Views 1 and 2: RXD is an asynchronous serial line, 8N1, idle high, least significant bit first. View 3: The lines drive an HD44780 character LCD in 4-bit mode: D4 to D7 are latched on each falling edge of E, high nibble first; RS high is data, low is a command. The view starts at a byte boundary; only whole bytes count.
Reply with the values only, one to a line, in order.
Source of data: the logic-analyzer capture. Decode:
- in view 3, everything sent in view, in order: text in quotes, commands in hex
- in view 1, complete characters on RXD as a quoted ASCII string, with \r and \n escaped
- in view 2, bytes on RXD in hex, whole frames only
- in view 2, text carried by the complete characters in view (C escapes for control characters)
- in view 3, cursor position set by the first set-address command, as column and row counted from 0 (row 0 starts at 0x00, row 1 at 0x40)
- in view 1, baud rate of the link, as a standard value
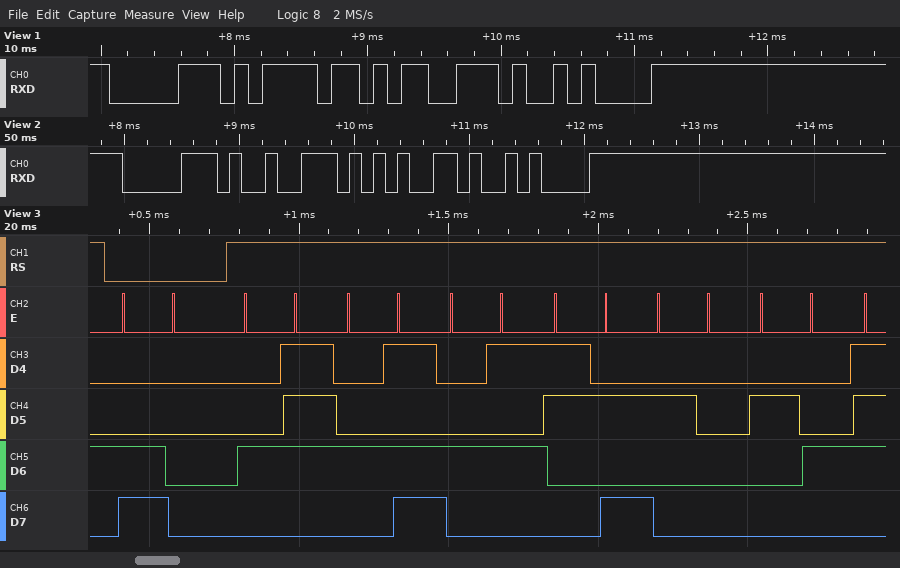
0xC0 "GME: $"
"pos\n"
70 72 65 0A
"pre\n"
column 0, row 1
9600 baud
